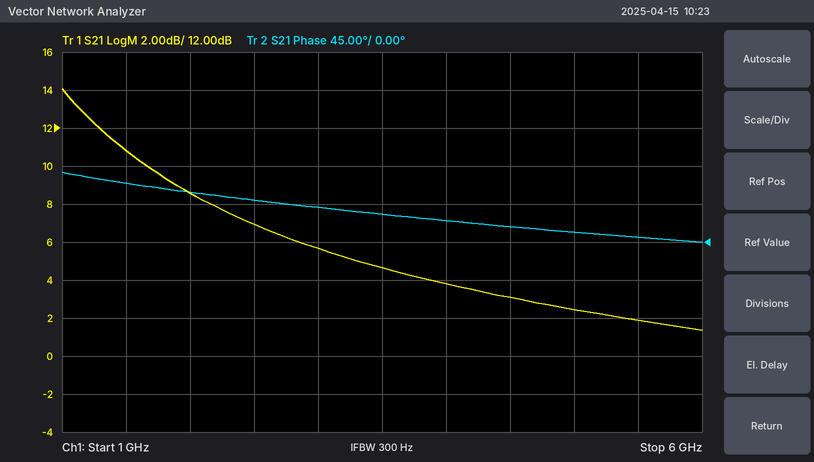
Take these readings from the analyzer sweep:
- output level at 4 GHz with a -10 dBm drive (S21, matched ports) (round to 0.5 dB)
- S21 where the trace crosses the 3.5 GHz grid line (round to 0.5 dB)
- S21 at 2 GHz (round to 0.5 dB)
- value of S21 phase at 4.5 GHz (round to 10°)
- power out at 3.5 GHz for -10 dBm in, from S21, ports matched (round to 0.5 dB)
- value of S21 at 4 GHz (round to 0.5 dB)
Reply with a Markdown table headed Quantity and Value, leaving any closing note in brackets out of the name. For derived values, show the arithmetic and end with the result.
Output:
| Quantity | Value |
|---|---|
| output level at 4 GHz with a -10 dBm drive (S21, matched ports) | -10 dBm + (4.0 dB) = -6.0 dBm |
| S21 where the trace crosses the 3.5 GHz grid line | 4.5 dB |
| S21 at 2 GHz | 8.5 dB |
| value of S21 phase at 4.5 GHz | 20° |
| power out at 3.5 GHz for -10 dBm in, from S21, ports matched | -10 dBm + (4.5 dB) = -5.5 dBm |
| value of S21 at 4 GHz | 4.0 dB |
